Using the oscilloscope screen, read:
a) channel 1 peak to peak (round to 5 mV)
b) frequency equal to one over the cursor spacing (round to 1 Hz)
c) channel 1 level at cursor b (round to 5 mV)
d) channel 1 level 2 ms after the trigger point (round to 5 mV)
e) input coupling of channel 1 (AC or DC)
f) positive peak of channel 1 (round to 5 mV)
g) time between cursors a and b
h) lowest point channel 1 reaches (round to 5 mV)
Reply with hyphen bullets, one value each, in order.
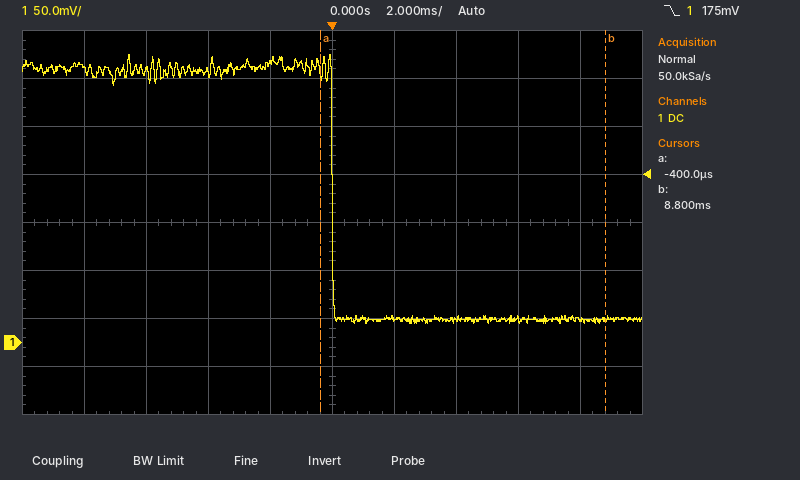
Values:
- 280 mV
- 109 Hz
- 25 mV
- 25 mV
- DC
- 300 mV
- 9.2 ms
- 20 mV
